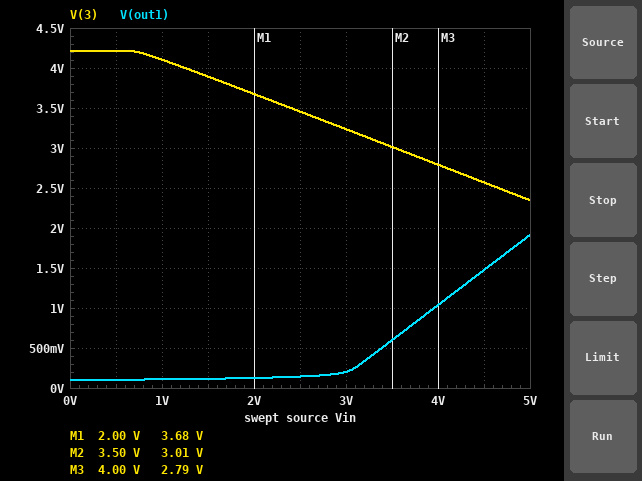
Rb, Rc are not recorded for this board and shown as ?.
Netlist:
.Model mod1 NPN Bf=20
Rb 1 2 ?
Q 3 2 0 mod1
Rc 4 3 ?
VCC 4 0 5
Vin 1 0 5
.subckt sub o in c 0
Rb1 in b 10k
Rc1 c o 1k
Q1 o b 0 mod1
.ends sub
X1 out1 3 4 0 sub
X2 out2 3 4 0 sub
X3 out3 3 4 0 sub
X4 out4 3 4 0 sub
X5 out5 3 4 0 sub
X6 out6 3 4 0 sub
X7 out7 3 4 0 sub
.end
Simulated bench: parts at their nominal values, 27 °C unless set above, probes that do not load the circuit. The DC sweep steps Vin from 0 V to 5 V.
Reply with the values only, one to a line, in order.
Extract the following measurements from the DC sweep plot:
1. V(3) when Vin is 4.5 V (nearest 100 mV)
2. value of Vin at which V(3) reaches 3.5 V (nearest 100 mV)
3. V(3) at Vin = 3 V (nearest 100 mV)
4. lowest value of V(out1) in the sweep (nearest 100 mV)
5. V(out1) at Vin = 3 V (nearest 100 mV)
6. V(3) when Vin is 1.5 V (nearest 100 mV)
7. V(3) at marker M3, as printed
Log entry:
2.6 V
2.4 V
3.2 V
100 mV
200 mV
3.9 V
2.79 V
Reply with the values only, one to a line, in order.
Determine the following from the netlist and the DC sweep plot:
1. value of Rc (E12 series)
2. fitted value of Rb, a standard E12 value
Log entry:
330 Ω
12 kΩ
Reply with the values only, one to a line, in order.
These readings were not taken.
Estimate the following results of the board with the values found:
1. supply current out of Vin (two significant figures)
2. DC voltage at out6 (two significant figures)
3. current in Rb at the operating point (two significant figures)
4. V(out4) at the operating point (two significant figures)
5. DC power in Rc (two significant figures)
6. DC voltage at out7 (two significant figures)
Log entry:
350 µA
1.9 V
350 µA
1.9 V
21 mW
1.9 V
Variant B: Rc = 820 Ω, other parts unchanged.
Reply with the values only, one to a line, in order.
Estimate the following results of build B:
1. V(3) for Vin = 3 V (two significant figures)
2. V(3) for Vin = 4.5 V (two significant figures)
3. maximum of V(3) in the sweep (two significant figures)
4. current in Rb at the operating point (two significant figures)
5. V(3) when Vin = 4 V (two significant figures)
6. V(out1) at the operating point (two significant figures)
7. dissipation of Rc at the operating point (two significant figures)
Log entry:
1.6 V
160 mV
3.5 V
350 µA
650 mV
5.0 V
29 mW
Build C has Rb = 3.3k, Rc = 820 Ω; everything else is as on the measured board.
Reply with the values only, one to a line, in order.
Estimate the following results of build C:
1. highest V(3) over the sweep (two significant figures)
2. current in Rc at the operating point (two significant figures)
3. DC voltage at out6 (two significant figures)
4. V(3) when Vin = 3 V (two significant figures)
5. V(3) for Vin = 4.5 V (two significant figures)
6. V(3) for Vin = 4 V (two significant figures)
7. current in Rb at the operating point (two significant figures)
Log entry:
3.5 V
6.0 mA
5.0 V
78 mV
60 mV
64 mV
1.3 mA
